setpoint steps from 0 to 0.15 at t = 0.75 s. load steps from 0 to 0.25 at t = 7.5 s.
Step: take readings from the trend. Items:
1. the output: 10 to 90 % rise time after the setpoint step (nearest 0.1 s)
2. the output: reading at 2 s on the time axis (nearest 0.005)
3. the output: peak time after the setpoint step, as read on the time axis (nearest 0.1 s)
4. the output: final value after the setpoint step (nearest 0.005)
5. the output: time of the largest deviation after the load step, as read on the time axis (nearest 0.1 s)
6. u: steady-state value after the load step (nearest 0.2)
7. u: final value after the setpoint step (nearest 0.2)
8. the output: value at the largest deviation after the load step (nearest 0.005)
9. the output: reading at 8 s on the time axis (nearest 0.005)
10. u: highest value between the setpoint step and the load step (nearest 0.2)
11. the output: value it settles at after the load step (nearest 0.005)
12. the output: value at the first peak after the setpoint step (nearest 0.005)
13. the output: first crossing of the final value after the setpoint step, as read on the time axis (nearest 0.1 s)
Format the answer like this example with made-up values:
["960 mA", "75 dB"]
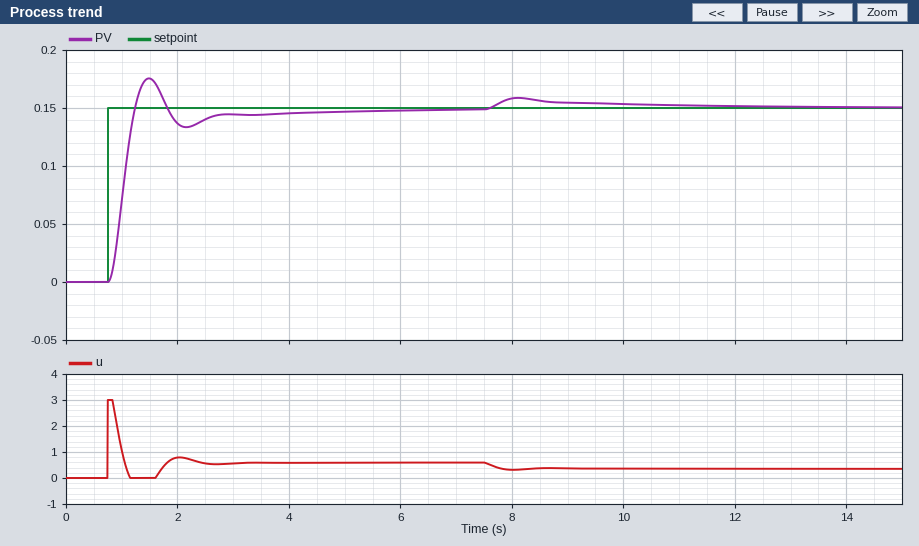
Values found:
["0.3 s", "0.135", "1.5 s", "0.150", "8.1 s", "0.4", "0.6", "0.160", "0.160", "3.0", "0.150", "0.175", "1.2 s"]
